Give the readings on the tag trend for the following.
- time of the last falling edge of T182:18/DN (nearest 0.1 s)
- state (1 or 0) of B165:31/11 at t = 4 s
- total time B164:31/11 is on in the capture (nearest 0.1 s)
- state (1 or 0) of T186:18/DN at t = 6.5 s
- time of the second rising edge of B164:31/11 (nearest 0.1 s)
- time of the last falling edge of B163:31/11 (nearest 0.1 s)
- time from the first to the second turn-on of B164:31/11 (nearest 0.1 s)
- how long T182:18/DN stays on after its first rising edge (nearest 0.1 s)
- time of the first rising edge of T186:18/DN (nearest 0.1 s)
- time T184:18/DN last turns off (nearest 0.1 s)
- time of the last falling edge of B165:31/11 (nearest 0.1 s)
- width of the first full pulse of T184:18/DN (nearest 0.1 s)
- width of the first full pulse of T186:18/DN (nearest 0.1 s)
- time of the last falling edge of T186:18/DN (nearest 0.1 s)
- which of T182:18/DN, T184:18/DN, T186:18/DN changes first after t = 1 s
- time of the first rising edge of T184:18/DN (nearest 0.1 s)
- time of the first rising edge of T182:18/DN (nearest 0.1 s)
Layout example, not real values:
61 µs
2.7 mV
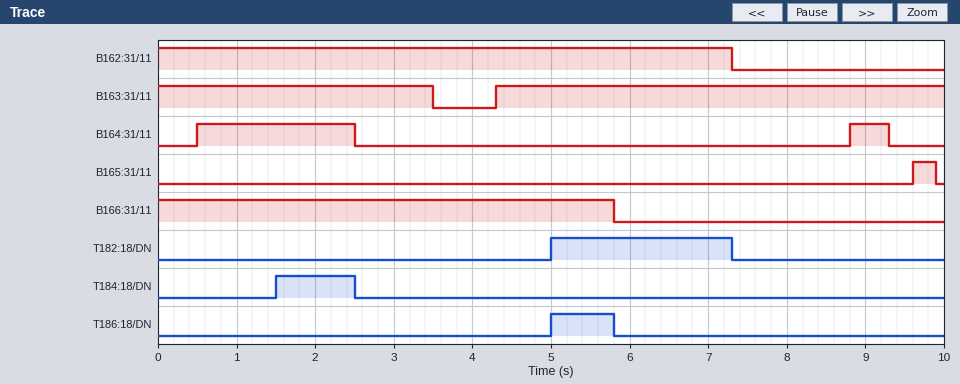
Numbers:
7.3 s
0
2.5 s
0
8.8 s
3.5 s
8.3 s
2.3 s
5.0 s
2.5 s
9.9 s
1.0 s
0.8 s
5.8 s
T184:18/DN
1.5 s
5.0 s
